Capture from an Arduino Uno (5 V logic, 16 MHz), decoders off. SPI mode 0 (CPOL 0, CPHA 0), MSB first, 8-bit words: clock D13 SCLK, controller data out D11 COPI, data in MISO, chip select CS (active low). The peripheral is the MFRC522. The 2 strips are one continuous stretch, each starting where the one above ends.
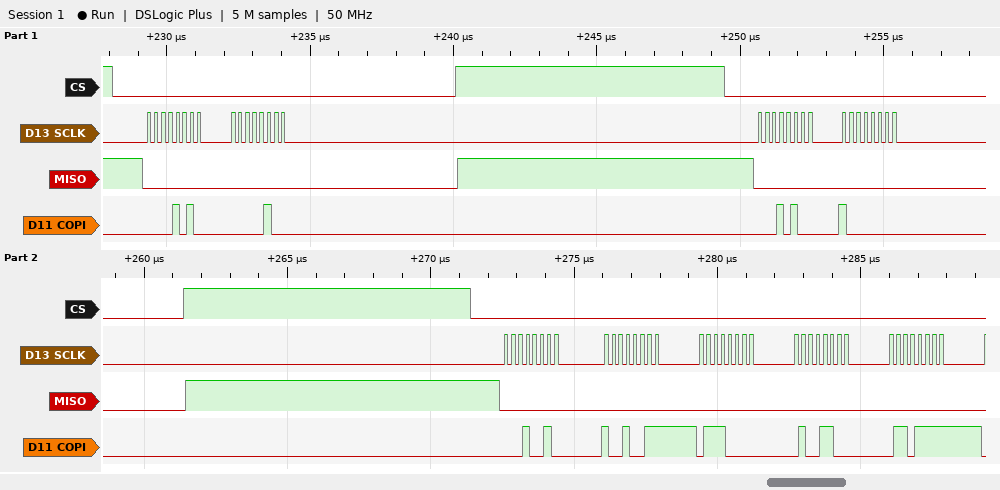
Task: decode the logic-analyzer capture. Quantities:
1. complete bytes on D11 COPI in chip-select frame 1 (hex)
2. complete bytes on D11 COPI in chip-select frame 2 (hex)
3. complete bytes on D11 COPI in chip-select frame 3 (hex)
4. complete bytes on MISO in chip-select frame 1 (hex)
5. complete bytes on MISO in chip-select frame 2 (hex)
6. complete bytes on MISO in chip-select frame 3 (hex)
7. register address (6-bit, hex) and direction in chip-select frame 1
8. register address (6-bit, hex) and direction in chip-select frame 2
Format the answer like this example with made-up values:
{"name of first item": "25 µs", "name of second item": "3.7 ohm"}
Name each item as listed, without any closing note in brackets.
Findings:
{"complete bytes on D11 COPI in chip-select frame 1": "0A 04", "complete bytes on D11 COPI in chip-select frame 2": "14 80", "complete bytes on D11 COPI in chip-select frame 3": "12 93 70 4C 6F", "complete bytes on MISO in chip-select frame 1": "00 00", "complete bytes on MISO in chip-select frame 2": "00 00", "complete bytes on MISO in chip-select frame 3": "00 00 00 00 00", "register address (6-bit, hex) and direction in chip-select frame 1": "0x05 write", "register address (6-bit, hex) and direction in chip-select frame 2": "0x0A write"}
